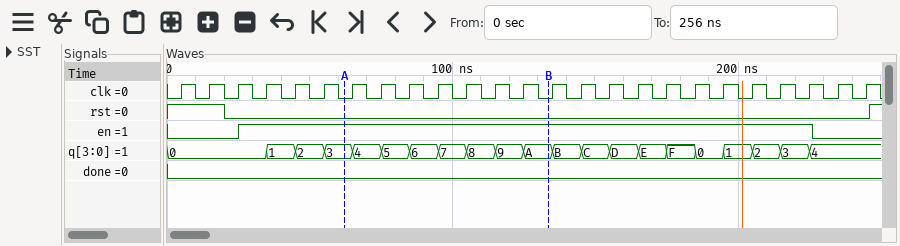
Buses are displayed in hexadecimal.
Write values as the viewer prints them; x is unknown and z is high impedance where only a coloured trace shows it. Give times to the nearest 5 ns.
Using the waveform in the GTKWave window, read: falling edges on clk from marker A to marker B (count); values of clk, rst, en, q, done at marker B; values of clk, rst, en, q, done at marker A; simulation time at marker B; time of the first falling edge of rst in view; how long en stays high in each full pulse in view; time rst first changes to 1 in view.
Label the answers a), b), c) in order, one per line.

a) 7
b) clk=0, rst=0, en=1, q=A, done=0
c) clk=0, rst=0, en=1, q=3, done=0
d) 135 ns
e) 20 ns
f) 200 ns
g) 245 ns
